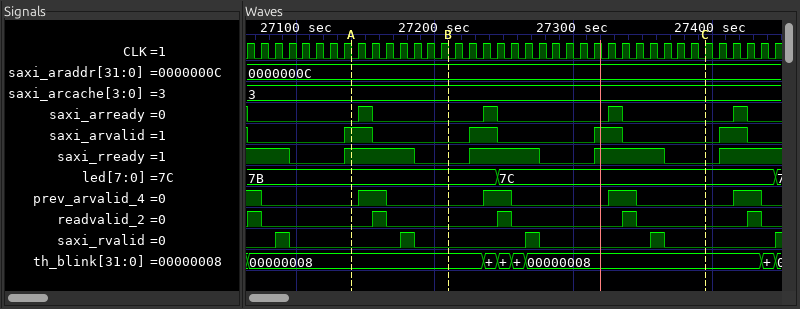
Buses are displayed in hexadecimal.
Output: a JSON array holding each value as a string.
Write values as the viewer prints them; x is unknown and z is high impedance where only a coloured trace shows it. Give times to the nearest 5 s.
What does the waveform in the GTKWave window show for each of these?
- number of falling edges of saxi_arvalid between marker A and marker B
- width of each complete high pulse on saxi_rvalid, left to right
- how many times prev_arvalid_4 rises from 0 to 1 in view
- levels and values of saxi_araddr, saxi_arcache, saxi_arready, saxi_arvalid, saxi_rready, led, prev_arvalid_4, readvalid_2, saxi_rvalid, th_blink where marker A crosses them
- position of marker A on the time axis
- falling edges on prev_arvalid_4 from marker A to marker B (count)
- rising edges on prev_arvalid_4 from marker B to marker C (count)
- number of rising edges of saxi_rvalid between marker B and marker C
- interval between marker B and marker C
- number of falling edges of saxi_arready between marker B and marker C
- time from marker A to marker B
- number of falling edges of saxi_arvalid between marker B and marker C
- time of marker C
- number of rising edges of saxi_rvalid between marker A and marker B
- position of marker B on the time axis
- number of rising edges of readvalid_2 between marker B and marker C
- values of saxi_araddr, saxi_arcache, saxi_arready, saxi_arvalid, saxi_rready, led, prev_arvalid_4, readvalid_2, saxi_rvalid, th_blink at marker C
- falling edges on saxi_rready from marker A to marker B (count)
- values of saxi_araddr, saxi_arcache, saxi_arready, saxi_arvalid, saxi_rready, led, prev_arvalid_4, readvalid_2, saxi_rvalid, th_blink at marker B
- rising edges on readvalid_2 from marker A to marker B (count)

["1", "10 s, 10 s, 10 s, 10 s", "4", "saxi_araddr=0000000C, saxi_arcache=3, saxi_arready=0, saxi_arvalid=1, saxi_rready=1, led=7B, prev_arvalid_4=0, readvalid_2=0, saxi_rvalid=0, th_blink=00000008", "27140 s", "1", "2", "2", "185 s", "2", "70 s", "2", "27395 s", "1", "27210 s", "2", "saxi_araddr=0000000C, saxi_arcache=3, saxi_arready=0, saxi_arvalid=0, saxi_rready=0, led=7C, prev_arvalid_4=0, readvalid_2=0, saxi_rvalid=0, th_blink=00000008", "1", "saxi_araddr=0000000C, saxi_arcache=3, saxi_arready=0, saxi_arvalid=0, saxi_rready=0, led=7B, prev_arvalid_4=0, readvalid_2=0, saxi_rvalid=0, th_blink=00000008", "1"]
